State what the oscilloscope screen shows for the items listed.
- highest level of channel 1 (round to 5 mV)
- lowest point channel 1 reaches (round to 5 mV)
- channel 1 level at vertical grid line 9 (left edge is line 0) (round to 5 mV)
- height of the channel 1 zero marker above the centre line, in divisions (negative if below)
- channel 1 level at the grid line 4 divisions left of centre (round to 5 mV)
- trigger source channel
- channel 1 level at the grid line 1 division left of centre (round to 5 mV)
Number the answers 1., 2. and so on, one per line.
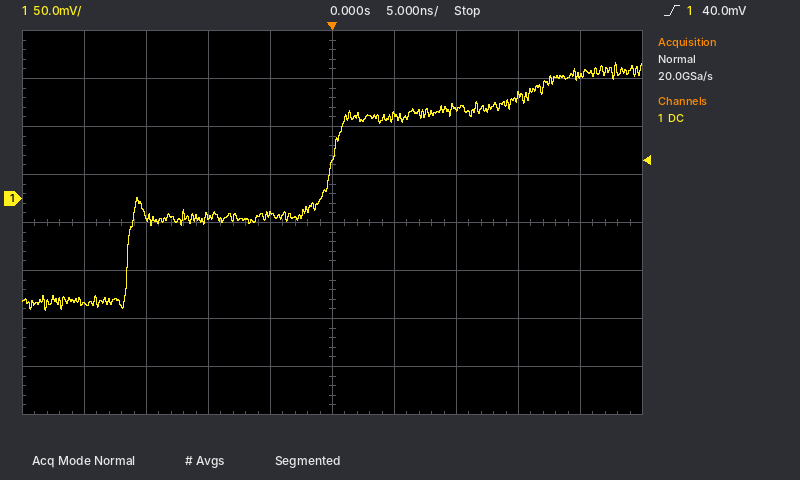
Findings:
1. 140 mV
2. -115 mV
3. 130 mV
4. +0.5 div
5. -110 mV
6. channel 1
7. -15 mV
